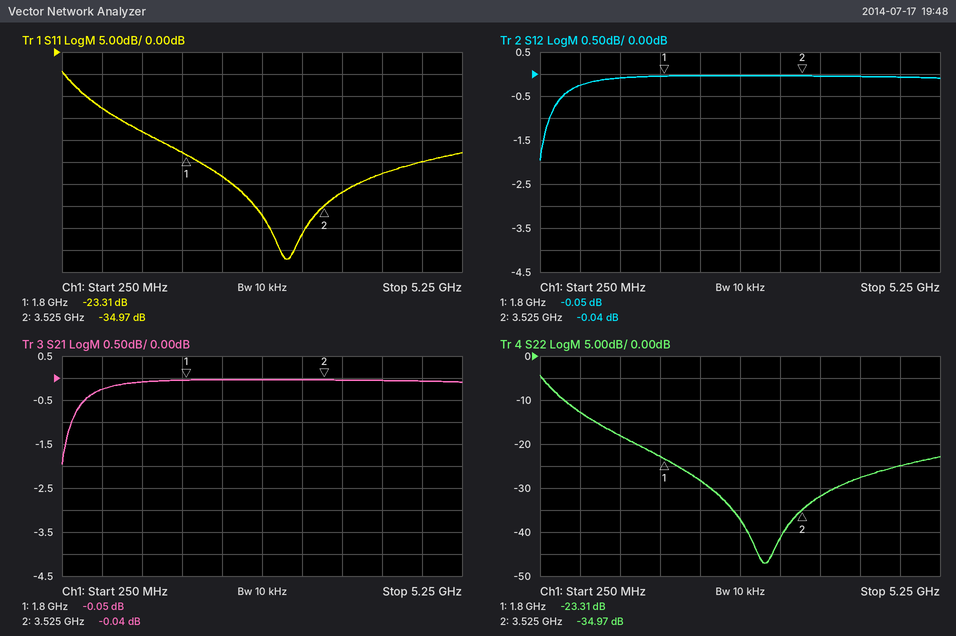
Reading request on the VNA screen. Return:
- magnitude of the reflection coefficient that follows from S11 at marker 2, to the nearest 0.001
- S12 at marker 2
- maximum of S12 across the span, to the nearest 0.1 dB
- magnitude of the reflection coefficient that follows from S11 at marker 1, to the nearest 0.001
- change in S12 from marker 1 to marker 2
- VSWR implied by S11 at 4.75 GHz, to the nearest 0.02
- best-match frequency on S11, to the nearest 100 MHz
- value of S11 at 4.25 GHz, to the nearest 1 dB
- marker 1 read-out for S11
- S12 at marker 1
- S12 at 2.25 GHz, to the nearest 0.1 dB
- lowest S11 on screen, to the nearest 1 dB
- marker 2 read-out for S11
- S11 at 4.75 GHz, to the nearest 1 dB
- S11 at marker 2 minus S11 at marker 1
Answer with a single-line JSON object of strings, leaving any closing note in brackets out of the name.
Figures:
{"magnitude of the reflection coefficient that follows from S11 at marker 2, to the nearest 0.001": "0.018", "S12 at marker 2": "-0.04 dB", "maximum of S12 across the span, to the nearest 0.1 dB": "0.0 dB", "magnitude of the reflection coefficient that follows from S11 at marker 1, to the nearest 0.001": "0.068", "change in S12 from marker 1 to marker 2": "0.01 dB", "VSWR implied by S11 at 4.75 GHz, to the nearest 0.02": "1.12", "best-match frequency on S11, to the nearest 100 MHz": "3.1 GHz", "value of S11 at 4.25 GHz, to the nearest 1 dB": "-28 dB", "marker 1 read-out for S11": "-23.31 dB", "S12 at marker 1": "-0.05 dB", "S12 at 2.25 GHz, to the nearest 0.1 dB": "0.0 dB", "lowest S11 on screen, to the nearest 1 dB": "-47 dB", "marker 2 read-out for S11": "-34.97 dB", "S11 at 4.75 GHz, to the nearest 1 dB": "-25 dB", "S11 at marker 2 minus S11 at marker 1": "-11.66 dB"}
